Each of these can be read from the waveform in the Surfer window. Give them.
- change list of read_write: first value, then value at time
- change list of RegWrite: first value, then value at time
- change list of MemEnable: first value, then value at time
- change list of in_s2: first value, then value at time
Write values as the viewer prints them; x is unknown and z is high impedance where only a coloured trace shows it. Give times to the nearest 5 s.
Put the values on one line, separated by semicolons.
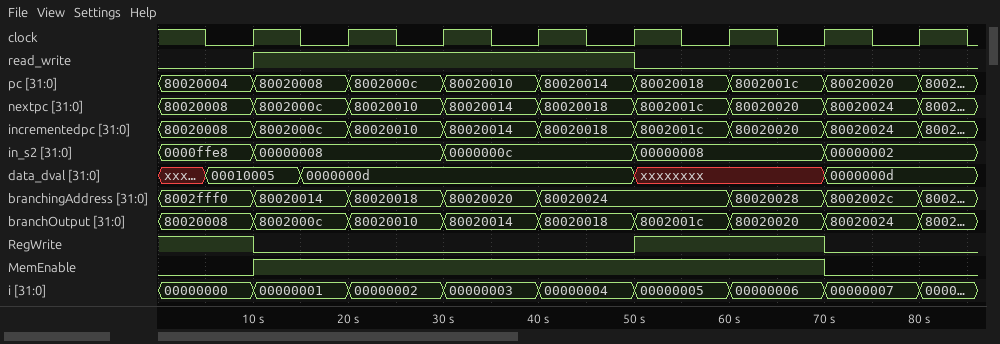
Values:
0, 1 at 10 s, 0 at 50 s; 1, 0 at 10 s, 1 at 50 s, 0 at 70 s; 0, 1 at 10 s, 0 at 70 s; 0000ffe8, 00000008 at 10 s, 0000000c at 30 s, 00000008 at 50 s, 00000002 at 70 s
